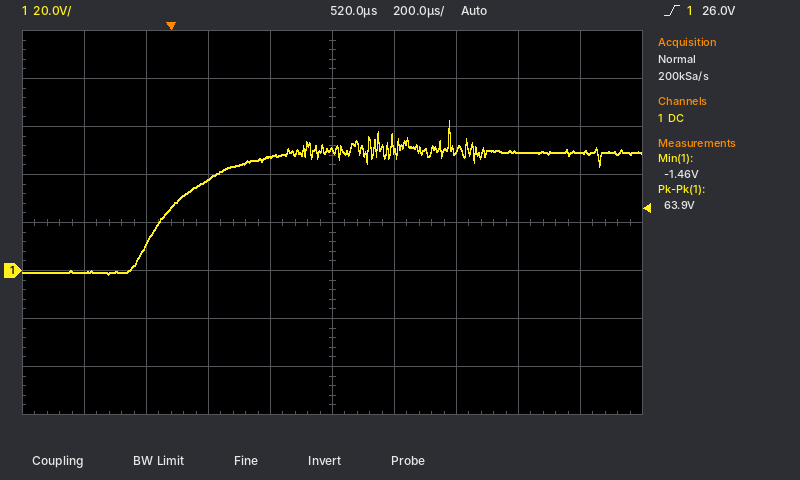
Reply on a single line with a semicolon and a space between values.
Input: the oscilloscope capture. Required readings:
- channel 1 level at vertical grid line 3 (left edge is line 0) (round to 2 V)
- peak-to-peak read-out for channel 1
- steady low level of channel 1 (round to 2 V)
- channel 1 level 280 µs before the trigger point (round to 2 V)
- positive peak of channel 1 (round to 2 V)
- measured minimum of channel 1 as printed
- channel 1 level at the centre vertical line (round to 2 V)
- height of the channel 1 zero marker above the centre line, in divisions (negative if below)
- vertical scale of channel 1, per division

38 V; 63.9 V; 0 V; 0 V; 62 V; -1.46 V; 50 V; -1.0 div; 20 V
